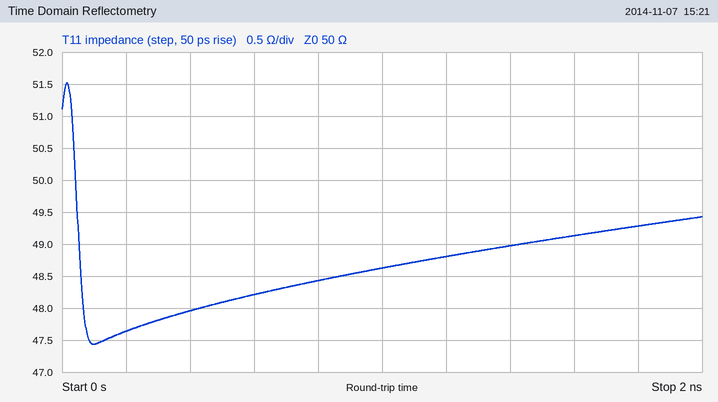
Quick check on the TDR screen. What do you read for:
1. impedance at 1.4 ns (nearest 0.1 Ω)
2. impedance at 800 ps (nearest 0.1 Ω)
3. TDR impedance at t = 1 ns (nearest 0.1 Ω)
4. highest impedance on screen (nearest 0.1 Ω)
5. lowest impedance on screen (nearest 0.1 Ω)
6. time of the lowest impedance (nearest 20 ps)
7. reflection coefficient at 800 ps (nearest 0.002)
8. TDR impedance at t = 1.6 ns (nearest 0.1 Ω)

49.0 Ω
48.4 Ω
48.6 Ω
51.5 Ω
47.4 Ω
100 ps
-0.016
49.1 Ω
